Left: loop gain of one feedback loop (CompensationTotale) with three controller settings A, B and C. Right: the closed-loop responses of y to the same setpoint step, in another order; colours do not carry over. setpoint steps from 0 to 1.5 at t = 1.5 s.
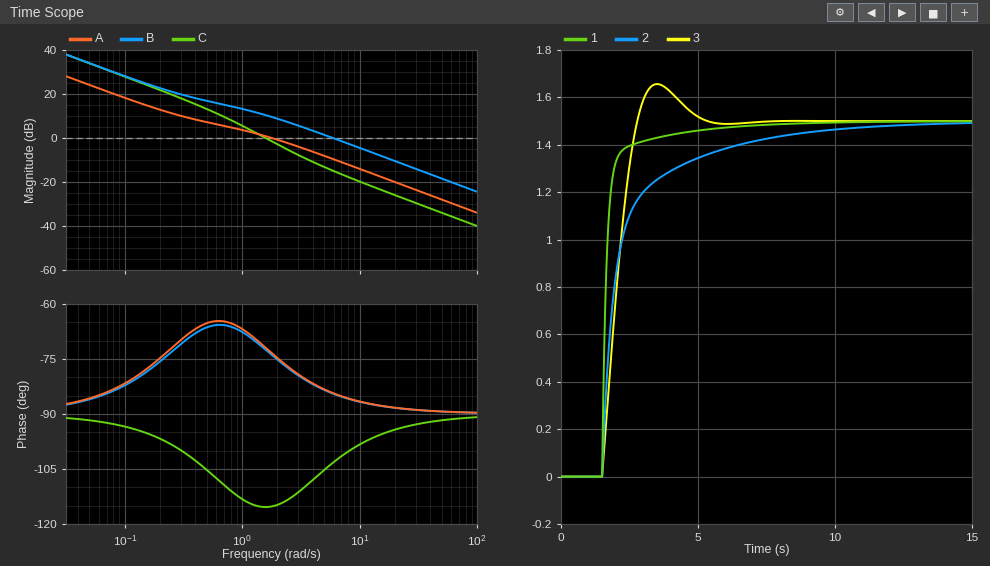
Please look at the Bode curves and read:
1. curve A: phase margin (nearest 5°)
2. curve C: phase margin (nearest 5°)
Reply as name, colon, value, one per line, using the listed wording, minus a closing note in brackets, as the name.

curve A: phase margin: 105°
curve C: phase margin: 65°
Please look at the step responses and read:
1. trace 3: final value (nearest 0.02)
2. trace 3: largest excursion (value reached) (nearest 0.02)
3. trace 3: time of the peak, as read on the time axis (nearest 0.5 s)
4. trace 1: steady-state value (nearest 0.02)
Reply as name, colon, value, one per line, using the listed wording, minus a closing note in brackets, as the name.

trace 3: final value: 1.50
trace 3: largest excursion (value reached): 1.66
trace 3: time of the peak, as read on the time axis: 3.5 s
trace 1: steady-state value: 1.50
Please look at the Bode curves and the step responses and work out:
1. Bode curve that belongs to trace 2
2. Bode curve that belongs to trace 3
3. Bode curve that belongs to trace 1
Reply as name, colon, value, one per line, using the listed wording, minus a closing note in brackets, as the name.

Bode curve that belongs to trace 2: A
Bode curve that belongs to trace 3: C
Bode curve that belongs to trace 1: B
